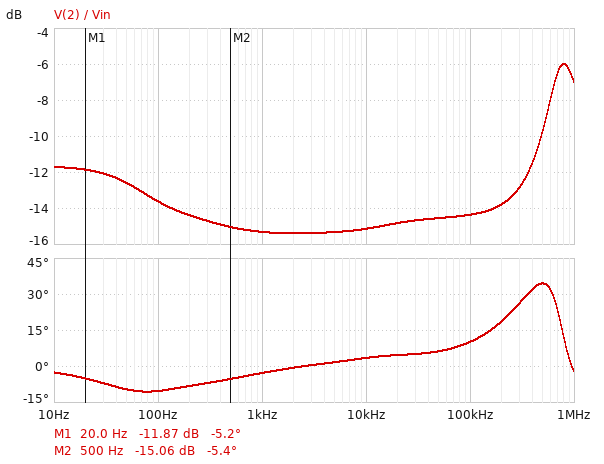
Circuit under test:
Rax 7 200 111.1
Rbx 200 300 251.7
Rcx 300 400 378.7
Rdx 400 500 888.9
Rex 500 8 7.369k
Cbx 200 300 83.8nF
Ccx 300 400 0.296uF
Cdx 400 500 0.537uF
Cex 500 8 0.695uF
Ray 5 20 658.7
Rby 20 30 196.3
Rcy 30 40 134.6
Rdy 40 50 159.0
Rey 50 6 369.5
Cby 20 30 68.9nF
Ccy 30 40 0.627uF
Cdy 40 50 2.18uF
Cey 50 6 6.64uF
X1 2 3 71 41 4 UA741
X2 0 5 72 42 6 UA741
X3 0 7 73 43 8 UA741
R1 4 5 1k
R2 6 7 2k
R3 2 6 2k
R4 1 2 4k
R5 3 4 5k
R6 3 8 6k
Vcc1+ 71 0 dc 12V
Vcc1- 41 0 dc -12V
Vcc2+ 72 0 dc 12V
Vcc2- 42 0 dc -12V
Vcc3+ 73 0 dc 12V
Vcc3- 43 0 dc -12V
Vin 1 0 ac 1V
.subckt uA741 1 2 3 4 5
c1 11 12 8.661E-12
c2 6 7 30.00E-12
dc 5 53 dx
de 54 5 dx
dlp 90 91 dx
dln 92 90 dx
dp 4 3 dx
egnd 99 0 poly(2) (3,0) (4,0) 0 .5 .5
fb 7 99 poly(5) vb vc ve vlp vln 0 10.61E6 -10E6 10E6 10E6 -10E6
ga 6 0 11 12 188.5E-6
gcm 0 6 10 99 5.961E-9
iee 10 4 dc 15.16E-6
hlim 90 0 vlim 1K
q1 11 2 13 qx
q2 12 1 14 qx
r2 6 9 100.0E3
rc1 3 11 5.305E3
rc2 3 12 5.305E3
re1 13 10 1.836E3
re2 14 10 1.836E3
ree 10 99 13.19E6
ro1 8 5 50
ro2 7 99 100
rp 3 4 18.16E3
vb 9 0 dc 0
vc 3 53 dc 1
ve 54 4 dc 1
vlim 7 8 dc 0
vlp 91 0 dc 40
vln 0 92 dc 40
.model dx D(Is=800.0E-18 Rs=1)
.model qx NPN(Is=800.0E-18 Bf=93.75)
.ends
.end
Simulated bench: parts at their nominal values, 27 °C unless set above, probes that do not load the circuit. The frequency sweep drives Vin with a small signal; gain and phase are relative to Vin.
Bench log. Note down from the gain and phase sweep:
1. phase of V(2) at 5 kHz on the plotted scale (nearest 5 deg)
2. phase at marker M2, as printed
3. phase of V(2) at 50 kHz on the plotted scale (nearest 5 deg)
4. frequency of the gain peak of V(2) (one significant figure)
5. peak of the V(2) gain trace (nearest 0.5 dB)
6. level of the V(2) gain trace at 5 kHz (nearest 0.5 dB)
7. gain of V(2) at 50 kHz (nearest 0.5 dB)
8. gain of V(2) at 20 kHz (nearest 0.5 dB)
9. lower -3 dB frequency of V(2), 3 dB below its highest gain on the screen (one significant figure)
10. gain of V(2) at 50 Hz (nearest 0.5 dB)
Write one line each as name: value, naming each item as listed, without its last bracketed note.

phase of V(2) at 5 kHz on the plotted scale: 0 deg
phase at marker M2, as printed: -5.4 deg
phase of V(2) at 50 kHz on the plotted scale: 5 deg
frequency of the gain peak of V(2): 800 kHz
peak of the V(2) gain trace: -6.0 dB
level of the V(2) gain trace at 5 kHz: -15.5 dB
gain of V(2) at 50 kHz: -14.5 dB
gain of V(2) at 20 kHz: -15.0 dB
lower -3 dB frequency of V(2), 3 dB below its highest gain on the screen: 500 kHz
gain of V(2) at 50 Hz: -12.5 dB
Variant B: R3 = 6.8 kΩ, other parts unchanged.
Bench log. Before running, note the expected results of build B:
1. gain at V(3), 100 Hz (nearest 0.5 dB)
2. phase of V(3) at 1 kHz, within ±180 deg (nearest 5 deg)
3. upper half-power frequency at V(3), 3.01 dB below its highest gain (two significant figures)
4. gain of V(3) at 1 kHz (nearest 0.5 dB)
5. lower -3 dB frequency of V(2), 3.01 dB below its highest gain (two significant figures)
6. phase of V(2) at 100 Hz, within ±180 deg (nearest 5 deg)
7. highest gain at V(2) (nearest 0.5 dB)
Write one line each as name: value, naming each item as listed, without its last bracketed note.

gain at V(3), 100 Hz: -6.5 dB
phase of V(3) at 1 kHz, within ±180 deg: 0 deg
upper half-power frequency at V(3), 3.01 dB below its highest gain: 960 kHz
gain of V(3) at 1 kHz: -7.5 dB
lower -3 dB frequency of V(2), 3.01 dB below its highest gain: 360 kHz
phase of V(2) at 100 Hz, within ±180 deg: -5 deg
highest gain at V(2): -2.0 dB
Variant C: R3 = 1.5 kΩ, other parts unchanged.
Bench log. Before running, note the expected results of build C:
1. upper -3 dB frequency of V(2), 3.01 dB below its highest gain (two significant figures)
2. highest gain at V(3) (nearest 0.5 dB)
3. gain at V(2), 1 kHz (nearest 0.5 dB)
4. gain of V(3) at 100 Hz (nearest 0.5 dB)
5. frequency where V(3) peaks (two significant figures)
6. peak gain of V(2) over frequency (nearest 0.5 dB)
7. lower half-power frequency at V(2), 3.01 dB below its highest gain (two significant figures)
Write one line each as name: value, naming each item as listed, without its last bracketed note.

upper -3 dB frequency of V(2), 3.01 dB below its highest gain: 1.4 MHz
highest gain at V(3): -11.0 dB
gain at V(2), 1 kHz: -17.5 dB
gain of V(3) at 100 Hz: -15.5 dB
frequency where V(3) peaks: 720 kHz
peak gain of V(2) over frequency: -7.5 dB
lower half-power frequency at V(2), 3.01 dB below its highest gain: 560 kHz
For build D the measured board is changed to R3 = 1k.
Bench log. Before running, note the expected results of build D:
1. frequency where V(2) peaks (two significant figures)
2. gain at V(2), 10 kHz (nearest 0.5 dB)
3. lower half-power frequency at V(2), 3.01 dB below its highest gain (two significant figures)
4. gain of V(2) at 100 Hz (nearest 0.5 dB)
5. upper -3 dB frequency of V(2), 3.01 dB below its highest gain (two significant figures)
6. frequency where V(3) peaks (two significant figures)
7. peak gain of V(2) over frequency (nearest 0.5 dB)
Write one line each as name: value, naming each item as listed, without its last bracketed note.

frequency where V(2) peaks: 810 kHz
gain at V(2), 10 kHz: -20.5 dB
lower half-power frequency at V(2), 3.01 dB below its highest gain: 590 kHz
gain of V(2) at 100 Hz: -18.5 dB
upper -3 dB frequency of V(2), 3.01 dB below its highest gain: 1.3 MHz
frequency where V(3) peaks: 740 kHz
peak gain of V(2) over frequency: -9.5 dB
